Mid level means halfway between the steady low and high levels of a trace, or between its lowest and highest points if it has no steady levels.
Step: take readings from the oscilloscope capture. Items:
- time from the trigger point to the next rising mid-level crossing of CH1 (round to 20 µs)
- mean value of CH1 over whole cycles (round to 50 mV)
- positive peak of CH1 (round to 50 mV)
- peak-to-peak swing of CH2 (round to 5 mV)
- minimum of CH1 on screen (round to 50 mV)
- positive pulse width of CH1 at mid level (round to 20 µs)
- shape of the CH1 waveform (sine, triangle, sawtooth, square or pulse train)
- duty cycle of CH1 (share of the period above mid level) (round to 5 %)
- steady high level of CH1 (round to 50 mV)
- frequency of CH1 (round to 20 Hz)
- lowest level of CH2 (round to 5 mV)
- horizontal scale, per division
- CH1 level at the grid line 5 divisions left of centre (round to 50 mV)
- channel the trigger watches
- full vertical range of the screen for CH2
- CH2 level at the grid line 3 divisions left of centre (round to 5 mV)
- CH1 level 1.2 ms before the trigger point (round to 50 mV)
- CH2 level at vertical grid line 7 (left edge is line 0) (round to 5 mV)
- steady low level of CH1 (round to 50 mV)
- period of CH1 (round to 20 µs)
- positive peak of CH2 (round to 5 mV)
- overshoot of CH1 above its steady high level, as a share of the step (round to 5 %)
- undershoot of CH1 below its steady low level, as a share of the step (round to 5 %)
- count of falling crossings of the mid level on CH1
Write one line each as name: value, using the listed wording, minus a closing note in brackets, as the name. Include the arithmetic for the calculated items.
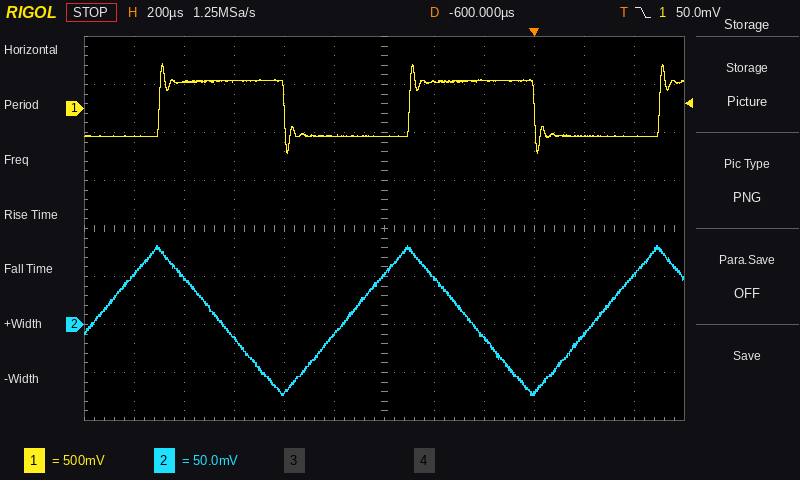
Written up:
time from the trigger point to the next rising mid-level crossing of CH1: 500 µs
mean value of CH1 over whole cycles: -300 mV + 0.5 × (300 mV − (-300 mV)) ≈ 0 mV
positive peak of CH1: 450 mV
peak-to-peak swing of CH2: 80 mV − (-75 mV) = 155 mV
minimum of CH1 on screen: -450 mV
positive pulse width of CH1 at mid level: 500 µs
shape of the CH1 waveform: square
duty cycle of CH1 (share of the period above mid level): 500 µs / 1.00 ms ≈ 50 %
steady high level of CH1: 300 mV
frequency of CH1: 1 / 1.00 ms ≈ 1.00 kHz
lowest level of CH2: -75 mV
horizontal scale, per division: 200 µs
CH1 level at the grid line 5 divisions left of centre: -300 mV
channel the trigger watches: CH1
full vertical range of the screen for CH2: 400 mV
CH2 level at the grid line 3 divisions left of centre: -15 mV
CH1 level 1.2 ms before the trigger point: 300 mV
CH2 level at vertical grid line 7 (left edge is line 0): 50 mV
steady low level of CH1: -300 mV
period of CH1: 1.00 ms
positive peak of CH2: 80 mV
overshoot of CH1 above its steady high level, as a share of the step: 30 %
undershoot of CH1 below its steady low level, as a share of the step: 30 %
count of falling crossings of the mid level on CH1: 2
